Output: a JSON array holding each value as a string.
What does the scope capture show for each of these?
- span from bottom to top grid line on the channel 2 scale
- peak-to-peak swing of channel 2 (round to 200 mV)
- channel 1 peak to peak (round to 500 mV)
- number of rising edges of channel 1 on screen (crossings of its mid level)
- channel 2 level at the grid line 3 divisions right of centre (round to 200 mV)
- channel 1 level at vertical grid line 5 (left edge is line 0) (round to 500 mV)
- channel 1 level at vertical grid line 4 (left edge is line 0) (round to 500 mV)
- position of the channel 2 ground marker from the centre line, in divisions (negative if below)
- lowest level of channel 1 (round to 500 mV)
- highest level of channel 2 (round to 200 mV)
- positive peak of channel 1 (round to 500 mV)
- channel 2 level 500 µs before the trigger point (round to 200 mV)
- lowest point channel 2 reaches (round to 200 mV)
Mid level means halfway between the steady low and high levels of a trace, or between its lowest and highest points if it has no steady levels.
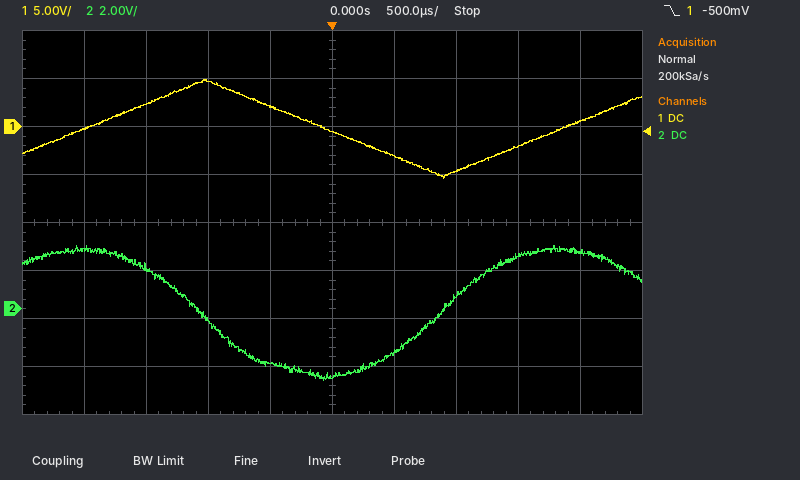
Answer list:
["16 V", "5.6 V", "10.5 V", "2", "2.2 V", "-500 mV", "2.0 V", "-1.8 div", "-5.5 V", "2.6 V", "5.0 V", "-2.2 V", "-3.0 V"]
